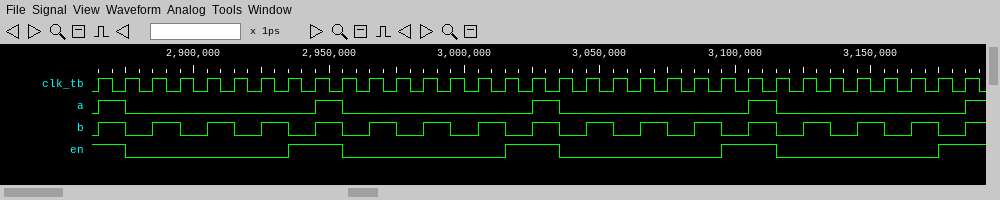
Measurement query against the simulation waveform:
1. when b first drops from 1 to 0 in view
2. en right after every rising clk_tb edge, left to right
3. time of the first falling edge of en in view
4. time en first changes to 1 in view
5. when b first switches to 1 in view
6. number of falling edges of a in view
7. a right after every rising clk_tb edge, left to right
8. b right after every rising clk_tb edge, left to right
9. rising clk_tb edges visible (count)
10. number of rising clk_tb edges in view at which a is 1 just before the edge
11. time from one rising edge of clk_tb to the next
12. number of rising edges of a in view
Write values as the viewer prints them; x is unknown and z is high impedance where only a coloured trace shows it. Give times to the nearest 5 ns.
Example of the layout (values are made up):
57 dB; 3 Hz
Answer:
2875 ns; 1 0 0 0 0 0 0 1 1 0 0 0 0 0 0 1 1 0 0 0 0 0 0 1 1 0 0 0 0 0 0 1 1; 2875 ns; 2935 ns; 2865 ns; 4; 1 0 0 0 0 0 0 0 1 0 0 0 0 0 0 0 1 0 0 0 0 0 0 0 1 0 0 0 0 0 0 0 1; 1 0 1 0 1 0 1 0 1 0 1 0 1 0 1 0 1 0 1 0 1 0 1 0 1 0 1 0 1 0 1 0 1; 33; 4; 10 ns; 5
